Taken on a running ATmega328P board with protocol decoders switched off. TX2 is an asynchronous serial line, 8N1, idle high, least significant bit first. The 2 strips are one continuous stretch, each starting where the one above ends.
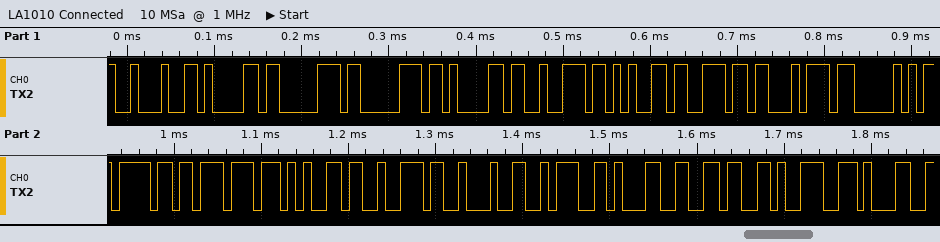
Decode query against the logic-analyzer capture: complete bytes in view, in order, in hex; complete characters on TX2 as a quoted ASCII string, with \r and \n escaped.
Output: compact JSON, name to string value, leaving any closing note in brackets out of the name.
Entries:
{"complete bytes in view, in order, in hex": "0x22 0x61 0x70 0x70 0x61 0x72 0x65 0x6E 0x74 0x50 0x6F 0x77 0x65 0x72 0x22 0x3A 0x31 0x36 0x39 0x31", "complete characters on TX2 as a quoted ASCII string, with \\r and \\n escaped": "\"\\\"apparentPower\\\":1691\""}
